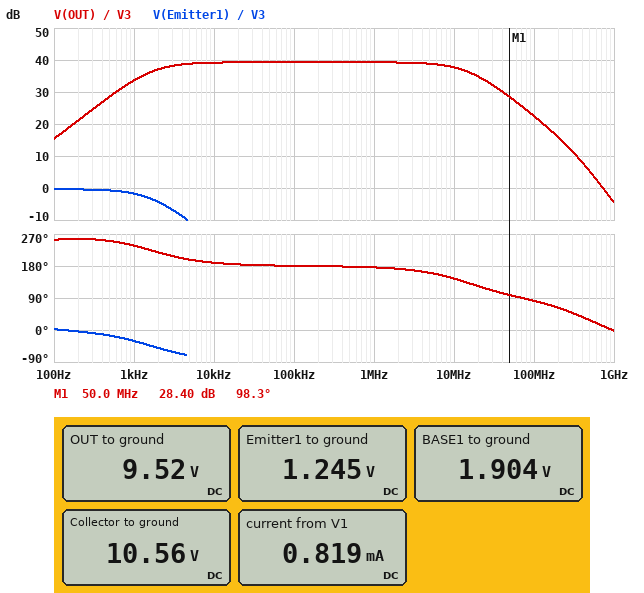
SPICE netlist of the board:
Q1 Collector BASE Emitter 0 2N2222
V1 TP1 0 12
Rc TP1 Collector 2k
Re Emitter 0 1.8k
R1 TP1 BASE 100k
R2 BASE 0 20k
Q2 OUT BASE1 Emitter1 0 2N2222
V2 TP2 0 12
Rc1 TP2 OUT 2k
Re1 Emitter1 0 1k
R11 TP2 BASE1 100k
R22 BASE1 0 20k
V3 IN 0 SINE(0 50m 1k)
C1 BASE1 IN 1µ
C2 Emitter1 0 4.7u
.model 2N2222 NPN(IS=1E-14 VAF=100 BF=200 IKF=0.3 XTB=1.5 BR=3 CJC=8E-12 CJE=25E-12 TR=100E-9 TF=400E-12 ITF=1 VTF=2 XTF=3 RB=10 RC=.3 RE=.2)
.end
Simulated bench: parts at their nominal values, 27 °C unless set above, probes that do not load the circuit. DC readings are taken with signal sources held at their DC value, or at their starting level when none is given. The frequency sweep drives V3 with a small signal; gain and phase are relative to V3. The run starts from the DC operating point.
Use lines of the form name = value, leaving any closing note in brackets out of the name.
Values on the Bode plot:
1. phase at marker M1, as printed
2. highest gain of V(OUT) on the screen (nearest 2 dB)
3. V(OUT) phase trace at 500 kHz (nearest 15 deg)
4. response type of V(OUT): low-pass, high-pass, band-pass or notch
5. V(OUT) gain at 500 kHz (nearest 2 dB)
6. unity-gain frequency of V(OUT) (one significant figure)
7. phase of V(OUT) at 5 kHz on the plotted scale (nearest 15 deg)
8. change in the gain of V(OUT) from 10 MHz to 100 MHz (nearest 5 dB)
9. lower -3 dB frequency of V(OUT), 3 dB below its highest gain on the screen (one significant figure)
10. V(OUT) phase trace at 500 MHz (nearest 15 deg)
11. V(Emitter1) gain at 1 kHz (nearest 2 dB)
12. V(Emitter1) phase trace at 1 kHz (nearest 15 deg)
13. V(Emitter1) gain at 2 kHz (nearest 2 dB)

phase at marker M1, as printed = 98.3 deg
highest gain of V(OUT) on the screen = 40 dB
V(OUT) phase trace at 500 kHz = 180 deg
response type of V(OUT): low-pass, high-pass, band-pass or notch = band-pass
V(OUT) gain at 500 kHz = 40 dB
unity-gain frequency of V(OUT) = 700 MHz
phase of V(OUT) at 5 kHz on the plotted scale = 195 deg
change in the gain of V(OUT) from 10 MHz to 100 MHz = -15 dB
lower -3 dB frequency of V(OUT), 3 dB below its highest gain on the screen = 2 kHz
V(OUT) phase trace at 500 MHz = 30 deg
V(Emitter1) gain at 1 kHz = -2 dB
V(Emitter1) phase trace at 1 kHz = -30 deg
V(Emitter1) gain at 2 kHz = -4 dB
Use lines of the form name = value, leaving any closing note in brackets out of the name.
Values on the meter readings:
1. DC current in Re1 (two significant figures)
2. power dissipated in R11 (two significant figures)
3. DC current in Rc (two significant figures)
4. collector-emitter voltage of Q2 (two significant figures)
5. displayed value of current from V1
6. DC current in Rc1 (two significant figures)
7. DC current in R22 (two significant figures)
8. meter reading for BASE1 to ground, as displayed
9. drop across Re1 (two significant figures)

DC current in Re1 = 1.2 mA
power dissipated in R11 = 1.0 mW
DC current in Rc = 720 µA
collector-emitter voltage of Q2 = 8.3 V
displayed value of current from V1 = 0.819 mA
DC current in Rc1 = 1.2 mA
DC current in R22 = 95 µA
meter reading for BASE1 to ground, as displayed = 1.904 V
drop across Re1 = 1.2 V
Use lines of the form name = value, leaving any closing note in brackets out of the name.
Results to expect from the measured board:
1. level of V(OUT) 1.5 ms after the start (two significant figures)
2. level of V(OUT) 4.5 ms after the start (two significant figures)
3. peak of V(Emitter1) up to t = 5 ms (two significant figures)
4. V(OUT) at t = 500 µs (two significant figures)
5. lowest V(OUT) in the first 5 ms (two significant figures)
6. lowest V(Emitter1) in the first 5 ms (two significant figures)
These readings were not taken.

level of V(OUT) 1.5 ms after the start = 11 V
level of V(OUT) 4.5 ms after the start = 11 V
peak of V(Emitter1) up to t = 5 ms = 1.3 V
V(OUT) at t = 500 µs = 11 V
lowest V(OUT) in the first 5 ms = 6.9 V
lowest V(Emitter1) in the first 5 ms = 1.2 V
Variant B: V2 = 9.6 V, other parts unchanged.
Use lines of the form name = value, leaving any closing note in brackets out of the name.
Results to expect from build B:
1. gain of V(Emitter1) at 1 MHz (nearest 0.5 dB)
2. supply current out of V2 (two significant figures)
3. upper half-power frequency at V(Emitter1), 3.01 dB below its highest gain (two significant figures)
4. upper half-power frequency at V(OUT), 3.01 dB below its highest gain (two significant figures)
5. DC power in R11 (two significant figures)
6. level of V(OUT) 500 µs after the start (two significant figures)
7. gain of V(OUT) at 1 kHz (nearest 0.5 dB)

gain of V(Emitter1) at 1 MHz = -59.0 dB
supply current out of V2 = 960 µA
upper half-power frequency at V(Emitter1), 3.01 dB below its highest gain = 1.2 kHz
upper half-power frequency at V(OUT), 3.01 dB below its highest gain = 16 MHz
DC power in R11 = 650 µW
level of V(OUT) 500 µs after the start = 9.0 V
gain of V(OUT) at 1 kHz = 32.5 dB
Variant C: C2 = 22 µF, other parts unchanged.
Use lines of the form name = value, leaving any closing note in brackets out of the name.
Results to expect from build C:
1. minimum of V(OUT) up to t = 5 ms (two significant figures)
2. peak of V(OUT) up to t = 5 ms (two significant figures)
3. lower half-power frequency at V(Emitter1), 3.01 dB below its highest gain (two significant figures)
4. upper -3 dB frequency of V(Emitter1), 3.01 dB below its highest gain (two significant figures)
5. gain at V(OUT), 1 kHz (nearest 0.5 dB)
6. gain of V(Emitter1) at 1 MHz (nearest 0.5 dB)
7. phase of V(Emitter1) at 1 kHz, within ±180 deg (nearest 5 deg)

minimum of V(OUT) up to t = 5 ms = 4.4 V
peak of V(OUT) up to t = 5 ms = 12 V
lower half-power frequency at V(Emitter1), 3.01 dB below its highest gain = 8.9 Hz
upper -3 dB frequency of V(Emitter1), 3.01 dB below its highest gain = 400 Hz
gain at V(OUT), 1 kHz = 38.5 dB
gain of V(Emitter1) at 1 MHz = -69.5 dB
phase of V(Emitter1) at 1 kHz, within ±180 deg = -70 deg
